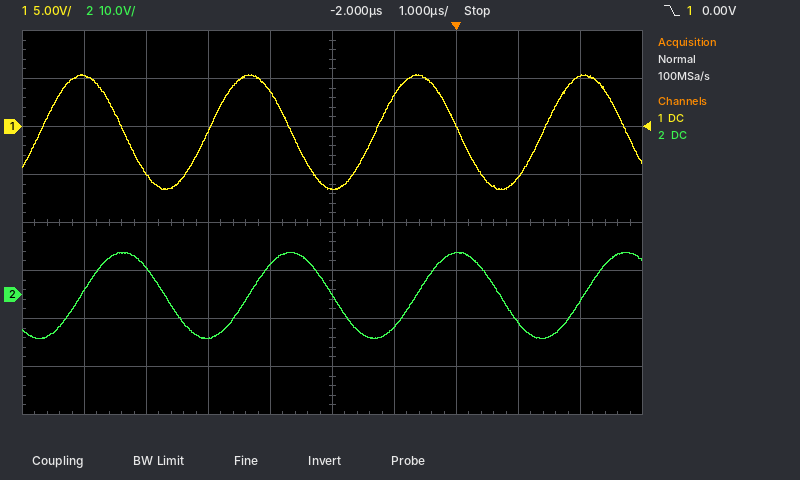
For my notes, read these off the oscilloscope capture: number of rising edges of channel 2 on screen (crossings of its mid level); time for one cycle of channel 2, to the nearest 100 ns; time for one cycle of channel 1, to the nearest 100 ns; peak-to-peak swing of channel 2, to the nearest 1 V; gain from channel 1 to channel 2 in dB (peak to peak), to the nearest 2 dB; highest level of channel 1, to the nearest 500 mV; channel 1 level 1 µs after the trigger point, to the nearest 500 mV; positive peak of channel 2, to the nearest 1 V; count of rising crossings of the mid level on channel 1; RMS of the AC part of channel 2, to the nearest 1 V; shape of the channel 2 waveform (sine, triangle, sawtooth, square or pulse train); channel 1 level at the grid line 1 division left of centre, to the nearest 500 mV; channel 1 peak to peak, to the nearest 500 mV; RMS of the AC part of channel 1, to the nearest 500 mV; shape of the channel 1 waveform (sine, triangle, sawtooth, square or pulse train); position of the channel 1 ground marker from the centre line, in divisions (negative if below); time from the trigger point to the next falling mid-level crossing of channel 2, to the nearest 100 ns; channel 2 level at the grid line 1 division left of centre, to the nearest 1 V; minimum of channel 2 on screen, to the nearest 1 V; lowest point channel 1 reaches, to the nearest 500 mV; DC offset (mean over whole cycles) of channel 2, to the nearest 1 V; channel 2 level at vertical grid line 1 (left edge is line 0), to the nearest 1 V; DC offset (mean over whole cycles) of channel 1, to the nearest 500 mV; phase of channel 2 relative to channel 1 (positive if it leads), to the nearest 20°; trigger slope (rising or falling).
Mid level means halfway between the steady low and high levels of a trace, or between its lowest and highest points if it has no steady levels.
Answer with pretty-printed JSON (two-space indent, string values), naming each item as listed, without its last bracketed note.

{
  "number of rising edges of channel 2 on screen": "4",
  "time for one cycle of channel 2, to the nearest 100 ns": "2.7 µs",
  "time for one cycle of channel 1, to the nearest 100 ns": "2.7 µs",
  "peak-to-peak swing of channel 2, to the nearest 1 V": "18 V",
  "gain from channel 1 to channel 2 in dB (peak to peak), to the nearest 2 dB": "4 dB",
  "highest level of channel 1, to the nearest 500 mV": "5.5 V",
  "channel 1 level 1 µs after the trigger point, to the nearest 500 mV": "-5.5 V",
  "positive peak of channel 2, to the nearest 1 V": "9 V",
  "count of rising crossings of the mid level on channel 1": "4",
  "RMS of the AC part of channel 2, to the nearest 1 V": "6 V",
  "shape of the channel 2 waveform": "sine",
  "channel 1 level at the grid line 1 division left of centre, to the nearest 500 mV": "3.5 V",
  "channel 1 peak to peak, to the nearest 500 mV": "12.0 V",
  "RMS of the AC part of channel 1, to the nearest 500 mV": "4.0 V",
  "shape of the channel 1 waveform": "sine",
  "position of the channel 1 ground marker from the centre line, in divisions": "+2.0 div",
  "time from the trigger point to the next falling mid-level crossing of channel 2, to the nearest 100 ns": "700 ns",
  "channel 2 level at the grid line 1 division left of centre, to the nearest 1 V": "6 V",
  "minimum of channel 2 on screen, to the nearest 1 V": "-9 V",
  "lowest point channel 1 reaches, to the nearest 500 mV": "-6.5 V",
  "DC offset (mean over whole cycles) of channel 2, to the nearest 1 V": "0 V",
  "channel 2 level at vertical grid line 1 (left edge is line 0), to the nearest 1 V": "1 V",
  "DC offset (mean over whole cycles) of channel 1, to the nearest 500 mV": "-500 mV",
  "phase of channel 2 relative to channel 1 (positive if it leads), to the nearest 20°": "-80°",
  "trigger slope": "falling"
}
